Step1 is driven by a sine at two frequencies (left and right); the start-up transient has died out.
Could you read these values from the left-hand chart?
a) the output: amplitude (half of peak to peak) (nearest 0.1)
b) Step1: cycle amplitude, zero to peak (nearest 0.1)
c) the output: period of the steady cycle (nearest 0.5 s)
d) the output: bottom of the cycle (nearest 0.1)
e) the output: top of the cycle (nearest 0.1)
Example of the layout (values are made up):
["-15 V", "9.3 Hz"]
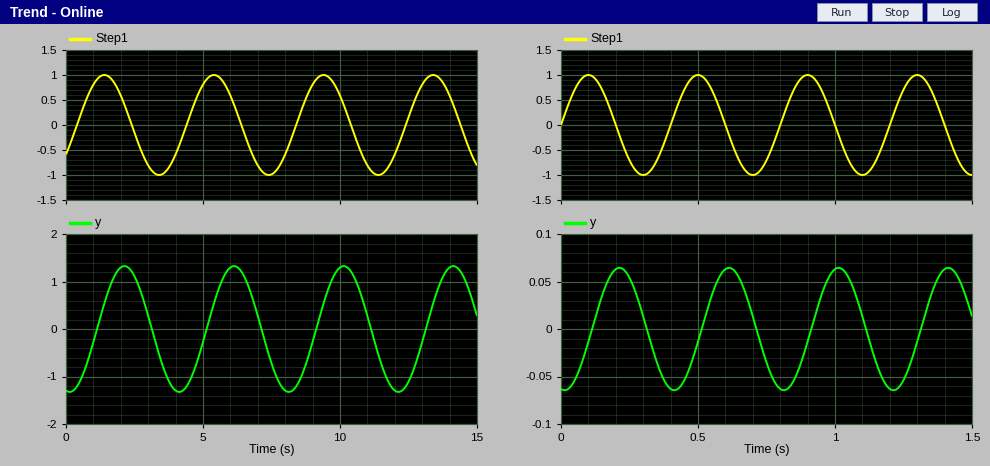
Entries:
["1.3", "1.0", "4.0 s", "-1.3", "1.3"]
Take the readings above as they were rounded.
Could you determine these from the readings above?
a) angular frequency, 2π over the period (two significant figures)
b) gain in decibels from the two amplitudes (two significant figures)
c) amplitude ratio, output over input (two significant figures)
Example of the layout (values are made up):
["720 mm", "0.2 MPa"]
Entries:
["1.6 rad/s", "2.3 dB", "1.3"]
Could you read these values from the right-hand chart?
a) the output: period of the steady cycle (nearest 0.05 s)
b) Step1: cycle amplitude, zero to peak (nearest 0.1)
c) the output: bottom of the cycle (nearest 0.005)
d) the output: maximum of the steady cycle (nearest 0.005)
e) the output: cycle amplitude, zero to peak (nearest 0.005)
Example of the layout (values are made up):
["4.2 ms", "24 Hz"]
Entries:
["0.40 s", "1.0", "-0.065", "0.065", "0.065"]
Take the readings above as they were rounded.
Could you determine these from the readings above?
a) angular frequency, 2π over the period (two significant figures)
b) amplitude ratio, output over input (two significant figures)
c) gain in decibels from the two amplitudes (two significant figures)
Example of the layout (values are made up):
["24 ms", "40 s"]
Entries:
["16 rad/s", "0.065", "-24 dB"]
